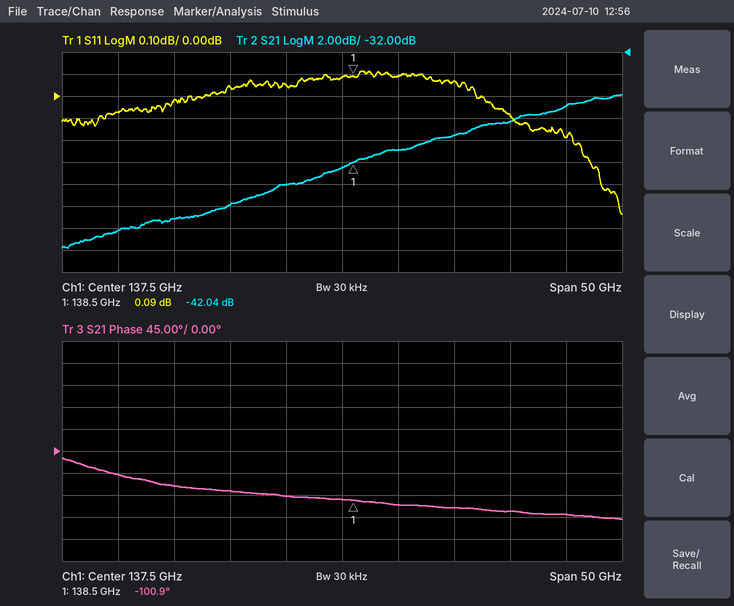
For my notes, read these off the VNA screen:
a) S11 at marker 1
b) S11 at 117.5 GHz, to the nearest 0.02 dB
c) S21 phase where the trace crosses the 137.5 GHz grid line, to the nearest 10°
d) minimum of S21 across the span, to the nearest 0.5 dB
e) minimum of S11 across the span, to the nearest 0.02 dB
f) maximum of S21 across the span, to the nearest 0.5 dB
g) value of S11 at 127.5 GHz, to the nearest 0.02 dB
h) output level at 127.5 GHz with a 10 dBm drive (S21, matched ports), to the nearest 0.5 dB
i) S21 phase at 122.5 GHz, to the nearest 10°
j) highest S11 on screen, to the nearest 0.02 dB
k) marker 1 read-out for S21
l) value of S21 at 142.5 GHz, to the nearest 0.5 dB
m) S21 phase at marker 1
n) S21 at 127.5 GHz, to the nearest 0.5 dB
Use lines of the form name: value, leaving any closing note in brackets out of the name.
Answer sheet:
S11 at marker 1: 0.09 dB
S11 at 117.5 GHz, to the nearest 0.02 dB: -0.08 dB
S21 phase where the trace crosses the 137.5 GHz grid line, to the nearest 10°: -100°
minimum of S21 across the span, to the nearest 0.5 dB: -50.0 dB
minimum of S11 across the span, to the nearest 0.02 dB: -0.54 dB
maximum of S21 across the span, to the nearest 0.5 dB: -36.0 dB
value of S11 at 127.5 GHz, to the nearest 0.02 dB: 0.04 dB
output level at 127.5 GHz with a 10 dBm drive (S21, matched ports), to the nearest 0.5 dB: -36.0 dBm
S21 phase at 122.5 GHz, to the nearest 10°: -70°
highest S11 on screen, to the nearest 0.02 dB: 0.12 dB
marker 1 read-out for S21: -42.04 dB
value of S21 at 142.5 GHz, to the nearest 0.5 dB: -41.0 dB
S21 phase at marker 1: -100.9°
S21 at 127.5 GHz, to the nearest 0.5 dB: -46.0 dB
